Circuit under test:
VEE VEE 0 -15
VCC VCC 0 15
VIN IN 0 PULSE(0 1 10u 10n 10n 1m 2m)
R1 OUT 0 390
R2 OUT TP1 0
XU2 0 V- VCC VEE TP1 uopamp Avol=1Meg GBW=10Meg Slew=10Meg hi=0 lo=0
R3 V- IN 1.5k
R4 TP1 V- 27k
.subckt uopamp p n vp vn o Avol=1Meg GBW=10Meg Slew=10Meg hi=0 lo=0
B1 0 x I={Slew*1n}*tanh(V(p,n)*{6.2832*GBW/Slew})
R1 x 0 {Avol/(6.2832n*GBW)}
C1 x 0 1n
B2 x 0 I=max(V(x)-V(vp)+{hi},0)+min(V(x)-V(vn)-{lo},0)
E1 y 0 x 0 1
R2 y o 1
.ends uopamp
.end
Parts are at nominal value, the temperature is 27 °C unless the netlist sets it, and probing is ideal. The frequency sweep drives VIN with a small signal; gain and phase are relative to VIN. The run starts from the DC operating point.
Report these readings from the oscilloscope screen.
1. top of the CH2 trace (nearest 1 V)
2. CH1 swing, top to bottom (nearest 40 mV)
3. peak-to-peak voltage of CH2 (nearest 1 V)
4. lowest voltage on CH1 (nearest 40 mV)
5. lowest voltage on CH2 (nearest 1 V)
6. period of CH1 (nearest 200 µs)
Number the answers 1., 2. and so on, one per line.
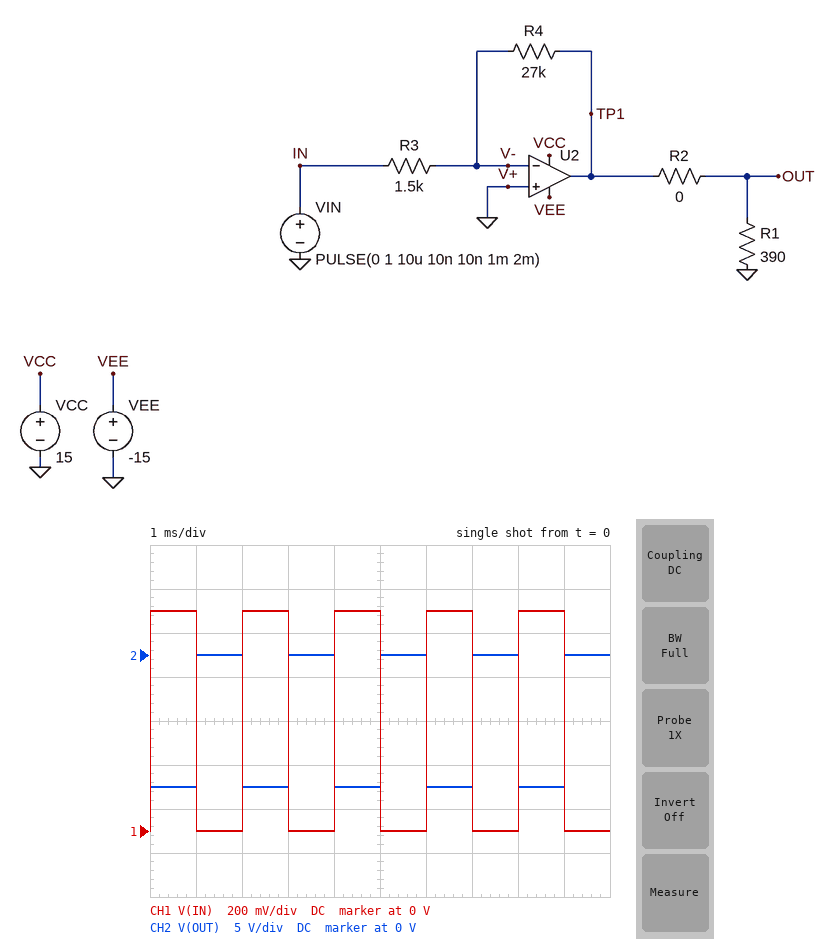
1. 0 V
2. 1.00 V
3. 15 V
4. 0 V
5. -15 V
6. 2.0 ms
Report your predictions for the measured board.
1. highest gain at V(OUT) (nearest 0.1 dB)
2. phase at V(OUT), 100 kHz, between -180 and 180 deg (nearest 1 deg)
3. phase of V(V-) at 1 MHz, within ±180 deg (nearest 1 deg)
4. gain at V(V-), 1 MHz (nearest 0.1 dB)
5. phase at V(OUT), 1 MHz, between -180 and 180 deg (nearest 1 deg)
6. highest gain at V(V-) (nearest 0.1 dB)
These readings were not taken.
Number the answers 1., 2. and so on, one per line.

1. 25.1 dB
2. 169 deg
3. 28 deg
4. -1.5 dB
5. 118 deg
6. -0.5 dB
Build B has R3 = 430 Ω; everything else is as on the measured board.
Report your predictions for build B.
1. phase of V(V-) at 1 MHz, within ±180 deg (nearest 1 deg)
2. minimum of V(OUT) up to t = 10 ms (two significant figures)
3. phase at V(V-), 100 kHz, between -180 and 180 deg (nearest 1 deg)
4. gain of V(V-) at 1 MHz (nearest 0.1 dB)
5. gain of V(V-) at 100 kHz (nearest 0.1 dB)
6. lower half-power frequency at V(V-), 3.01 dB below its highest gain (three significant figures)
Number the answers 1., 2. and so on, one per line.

1. 9 deg
2. -15 V
3. 57 deg
4. -0.2 dB
5. -5.5 dB
6. 156 kHz
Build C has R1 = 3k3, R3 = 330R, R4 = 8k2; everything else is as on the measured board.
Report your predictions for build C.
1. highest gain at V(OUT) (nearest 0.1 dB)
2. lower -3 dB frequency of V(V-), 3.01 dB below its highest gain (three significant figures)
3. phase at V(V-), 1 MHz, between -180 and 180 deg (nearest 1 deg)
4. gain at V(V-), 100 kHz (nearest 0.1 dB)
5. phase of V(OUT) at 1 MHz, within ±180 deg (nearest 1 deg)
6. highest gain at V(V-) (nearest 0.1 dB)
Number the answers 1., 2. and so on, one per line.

1. 27.9 dB
2. 387 kHz
3. 21 deg
4. -12.4 dB
5. 111 deg
6. -0.3 dB
